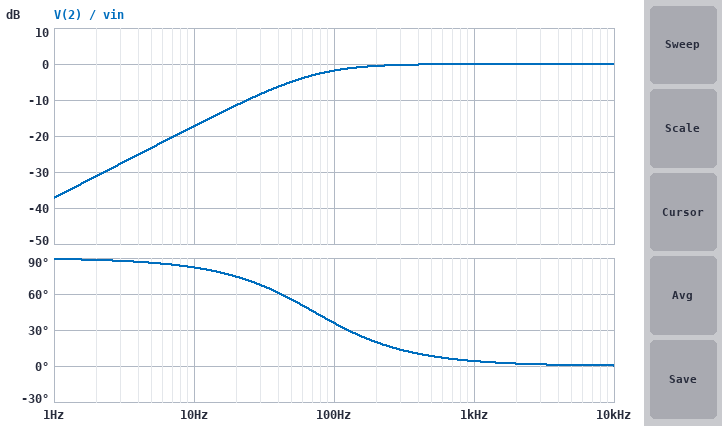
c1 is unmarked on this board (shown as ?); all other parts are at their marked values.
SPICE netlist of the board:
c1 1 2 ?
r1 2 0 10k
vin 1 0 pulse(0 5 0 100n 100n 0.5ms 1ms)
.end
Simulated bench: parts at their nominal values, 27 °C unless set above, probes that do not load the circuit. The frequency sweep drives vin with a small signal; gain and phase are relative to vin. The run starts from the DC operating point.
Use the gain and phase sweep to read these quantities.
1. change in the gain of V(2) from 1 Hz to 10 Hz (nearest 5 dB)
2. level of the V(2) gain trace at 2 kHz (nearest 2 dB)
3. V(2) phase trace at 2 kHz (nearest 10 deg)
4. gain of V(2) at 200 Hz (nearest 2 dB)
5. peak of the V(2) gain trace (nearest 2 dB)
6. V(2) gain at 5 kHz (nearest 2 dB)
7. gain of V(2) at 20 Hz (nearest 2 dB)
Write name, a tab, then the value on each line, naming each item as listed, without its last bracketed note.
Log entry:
change in the gain of V(2) from 1 Hz to 10 Hz	20 dB
level of the V(2) gain trace at 2 kHz	0 dB
V(2) phase trace at 2 kHz	0 deg
gain of V(2) at 200 Hz	0 dB
peak of the V(2) gain trace	0 dB
V(2) gain at 5 kHz	0 dB
gain of V(2) at 20 Hz	-12 dB
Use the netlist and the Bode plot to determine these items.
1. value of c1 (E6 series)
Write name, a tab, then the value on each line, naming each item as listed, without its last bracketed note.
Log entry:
value of c1	220 nF
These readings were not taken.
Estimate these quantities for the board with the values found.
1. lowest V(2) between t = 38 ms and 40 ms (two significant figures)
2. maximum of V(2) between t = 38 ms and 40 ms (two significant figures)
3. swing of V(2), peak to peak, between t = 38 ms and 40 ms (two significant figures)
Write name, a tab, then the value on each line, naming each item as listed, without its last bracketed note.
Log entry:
lowest V(2) between t = 38 ms and 40 ms	-2.8 V
maximum of V(2) between t = 38 ms and 40 ms	2.8 V
swing of V(2), peak to peak, between t = 38 ms and 40 ms	5.6 V
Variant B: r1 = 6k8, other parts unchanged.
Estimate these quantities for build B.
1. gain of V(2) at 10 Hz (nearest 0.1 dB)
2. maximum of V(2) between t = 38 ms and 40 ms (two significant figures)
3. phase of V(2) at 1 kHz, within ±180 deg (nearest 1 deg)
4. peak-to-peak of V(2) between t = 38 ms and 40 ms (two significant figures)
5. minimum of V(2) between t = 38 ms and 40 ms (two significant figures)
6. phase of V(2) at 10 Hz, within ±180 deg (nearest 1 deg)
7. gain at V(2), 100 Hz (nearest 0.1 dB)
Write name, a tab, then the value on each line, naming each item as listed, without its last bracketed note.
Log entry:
gain of V(2) at 10 Hz	-20.6 dB
maximum of V(2) between t = 38 ms and 40 ms	2.9 V
phase of V(2) at 1 kHz, within ±180 deg	6 deg
peak-to-peak of V(2) between t = 38 ms and 40 ms	5.8 V
minimum of V(2) between t = 38 ms and 40 ms	-2.9 V
phase of V(2) at 10 Hz, within ±180 deg	85 deg
gain at V(2), 100 Hz	-3.3 dB
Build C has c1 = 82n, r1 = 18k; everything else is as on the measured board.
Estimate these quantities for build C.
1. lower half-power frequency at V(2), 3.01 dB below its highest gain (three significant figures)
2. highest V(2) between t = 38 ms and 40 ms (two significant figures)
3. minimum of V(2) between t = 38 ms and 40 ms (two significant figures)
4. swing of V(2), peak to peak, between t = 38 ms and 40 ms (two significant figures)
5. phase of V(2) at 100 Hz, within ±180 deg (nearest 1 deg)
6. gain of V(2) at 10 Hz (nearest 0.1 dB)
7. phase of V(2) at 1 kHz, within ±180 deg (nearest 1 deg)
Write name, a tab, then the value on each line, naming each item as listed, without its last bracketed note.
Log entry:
lower half-power frequency at V(2), 3.01 dB below its highest gain	108 Hz
highest V(2) between t = 38 ms and 40 ms	2.9 V
minimum of V(2) between t = 38 ms and 40 ms	-2.9 V
swing of V(2), peak to peak, between t = 38 ms and 40 ms	5.8 V
phase of V(2) at 100 Hz, within ±180 deg	47 deg
gain of V(2) at 10 Hz	-20.7 dB
phase of V(2) at 1 kHz, within ±180 deg	6 deg
